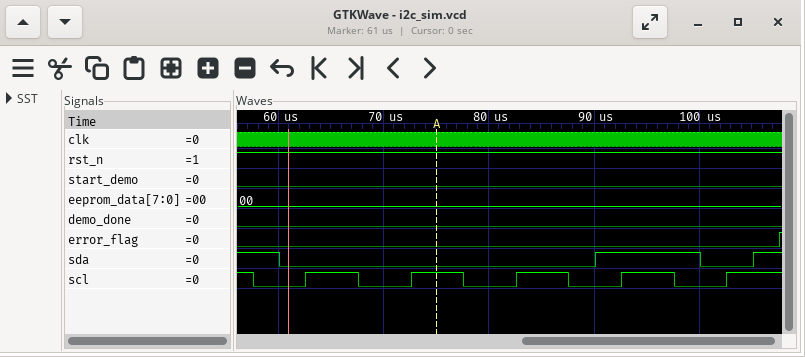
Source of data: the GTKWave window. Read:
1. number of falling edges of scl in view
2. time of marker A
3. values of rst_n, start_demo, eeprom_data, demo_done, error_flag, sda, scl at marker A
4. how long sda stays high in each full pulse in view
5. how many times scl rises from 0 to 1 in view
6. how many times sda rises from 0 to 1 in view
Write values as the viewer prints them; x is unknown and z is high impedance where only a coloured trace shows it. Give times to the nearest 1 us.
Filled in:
5
75 us
rst_n=1, start_demo=0, eeprom_data=00, demo_done=0, error_flag=0, sda=0, scl=1
10 us
5
2
